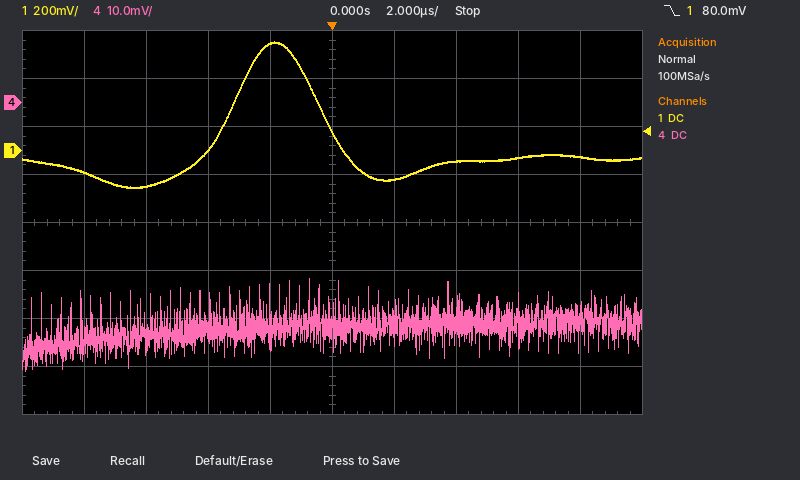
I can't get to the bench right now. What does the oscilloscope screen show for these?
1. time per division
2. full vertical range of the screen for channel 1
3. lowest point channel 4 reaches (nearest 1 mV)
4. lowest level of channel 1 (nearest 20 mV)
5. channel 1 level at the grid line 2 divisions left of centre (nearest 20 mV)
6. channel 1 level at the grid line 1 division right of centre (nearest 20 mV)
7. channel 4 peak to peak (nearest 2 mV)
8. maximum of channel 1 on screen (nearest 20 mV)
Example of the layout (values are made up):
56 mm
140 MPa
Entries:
2 µs
1.6 V
-56 mV
-160 mV
0 mV
-120 mV
20 mV
460 mV
